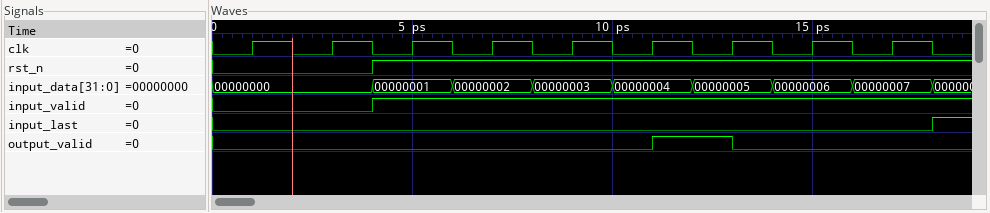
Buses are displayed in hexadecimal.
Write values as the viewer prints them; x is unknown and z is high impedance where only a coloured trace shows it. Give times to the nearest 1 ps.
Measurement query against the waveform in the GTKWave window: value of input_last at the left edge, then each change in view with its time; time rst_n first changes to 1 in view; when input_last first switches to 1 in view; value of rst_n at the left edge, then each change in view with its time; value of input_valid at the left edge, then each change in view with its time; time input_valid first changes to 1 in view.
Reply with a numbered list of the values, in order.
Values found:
1. 0, 1 at 18 ps
2. 4 ps
3. 18 ps
4. 0, 1 at 4 ps
5. 0, 1 at 4 ps
6. 4 ps
